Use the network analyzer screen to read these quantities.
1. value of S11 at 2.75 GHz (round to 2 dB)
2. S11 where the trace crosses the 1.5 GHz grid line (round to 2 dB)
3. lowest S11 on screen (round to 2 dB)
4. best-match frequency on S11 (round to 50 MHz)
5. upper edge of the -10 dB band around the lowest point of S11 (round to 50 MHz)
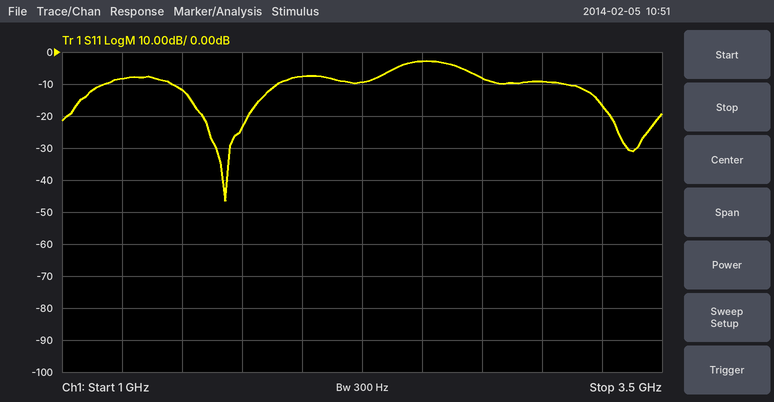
-8 dB
-12 dB
-46 dB
1.70 GHz
1.90 GHz
